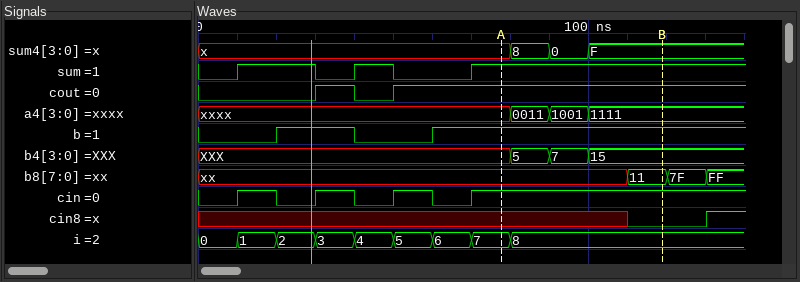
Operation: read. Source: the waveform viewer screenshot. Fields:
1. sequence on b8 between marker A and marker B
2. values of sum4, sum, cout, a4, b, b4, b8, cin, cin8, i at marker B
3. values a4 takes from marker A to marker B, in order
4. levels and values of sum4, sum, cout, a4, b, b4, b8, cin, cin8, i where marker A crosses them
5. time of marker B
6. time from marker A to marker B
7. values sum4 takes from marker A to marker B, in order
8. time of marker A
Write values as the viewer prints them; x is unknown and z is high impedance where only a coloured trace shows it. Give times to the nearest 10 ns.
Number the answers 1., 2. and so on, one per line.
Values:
1. xx, 11
2. sum4=F, sum=1, cout=1, a4=1111, b=1, b4=15, b8=11, cin=1, cin8=0, i=8
3. xxxx, 0011, 1001, 1111
4. sum4=x, sum=1, cout=1, a4=xxxx, b=1, b4=XXX, b8=xx, cin=1, cin8=x, i=7
5. 120 ns
6. 40 ns
7. x, 8, 0, F
8. 80 ns
